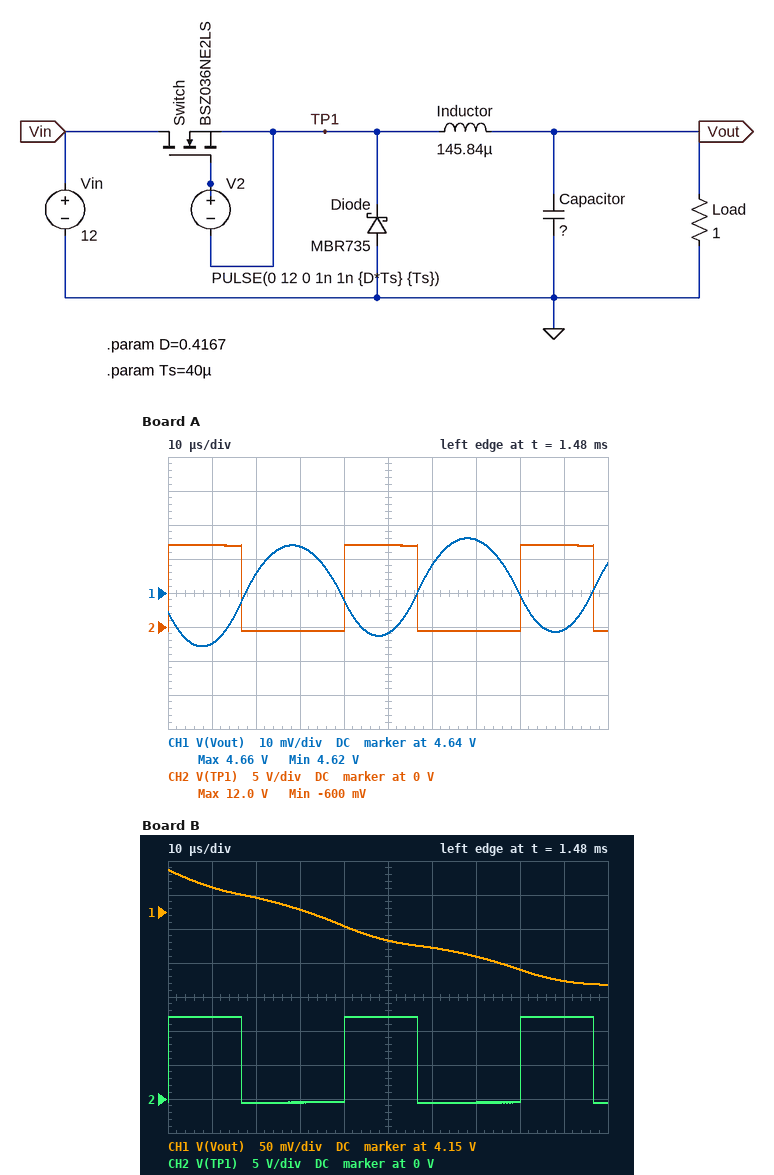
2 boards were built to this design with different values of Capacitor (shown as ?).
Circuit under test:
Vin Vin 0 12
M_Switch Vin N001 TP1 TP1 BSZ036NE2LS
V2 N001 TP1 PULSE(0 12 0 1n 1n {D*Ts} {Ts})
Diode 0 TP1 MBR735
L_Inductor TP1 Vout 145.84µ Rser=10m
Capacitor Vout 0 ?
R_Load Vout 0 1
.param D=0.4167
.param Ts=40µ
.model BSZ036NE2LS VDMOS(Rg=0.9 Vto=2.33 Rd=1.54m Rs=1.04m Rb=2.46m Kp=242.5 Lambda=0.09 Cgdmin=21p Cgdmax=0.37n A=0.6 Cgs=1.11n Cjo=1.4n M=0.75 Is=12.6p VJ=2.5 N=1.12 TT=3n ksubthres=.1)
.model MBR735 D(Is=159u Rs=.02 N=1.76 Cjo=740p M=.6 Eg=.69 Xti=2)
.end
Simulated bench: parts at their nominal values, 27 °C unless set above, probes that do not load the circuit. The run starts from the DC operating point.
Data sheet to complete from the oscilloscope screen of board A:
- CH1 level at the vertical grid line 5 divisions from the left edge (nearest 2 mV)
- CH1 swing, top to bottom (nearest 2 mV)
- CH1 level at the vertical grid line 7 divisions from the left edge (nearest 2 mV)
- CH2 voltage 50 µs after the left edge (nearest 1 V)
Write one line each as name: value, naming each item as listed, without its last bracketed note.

CH1 level at the vertical grid line 5 divisions from the left edge: 4.628 V
CH1 swing, top to bottom: 32 mV
CH1 level at the vertical grid line 7 divisions from the left edge: 4.656 V
CH2 voltage 50 µs after the left edge: 12 V
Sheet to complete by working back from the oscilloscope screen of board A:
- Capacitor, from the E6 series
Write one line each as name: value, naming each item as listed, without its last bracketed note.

Capacitor, from the E6 series: 150 µF
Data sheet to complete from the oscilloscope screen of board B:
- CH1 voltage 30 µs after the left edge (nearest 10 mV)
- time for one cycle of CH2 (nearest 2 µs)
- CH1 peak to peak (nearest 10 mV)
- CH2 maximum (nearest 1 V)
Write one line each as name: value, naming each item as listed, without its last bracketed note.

CH1 voltage 30 µs after the left edge: 4.15 V
time for one cycle of CH2: 40 µs
CH1 peak to peak: 170 mV
CH2 maximum: 12 V
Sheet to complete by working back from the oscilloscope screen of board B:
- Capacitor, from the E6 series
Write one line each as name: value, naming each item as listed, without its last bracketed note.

Capacitor, from the E6 series: 470 µF
